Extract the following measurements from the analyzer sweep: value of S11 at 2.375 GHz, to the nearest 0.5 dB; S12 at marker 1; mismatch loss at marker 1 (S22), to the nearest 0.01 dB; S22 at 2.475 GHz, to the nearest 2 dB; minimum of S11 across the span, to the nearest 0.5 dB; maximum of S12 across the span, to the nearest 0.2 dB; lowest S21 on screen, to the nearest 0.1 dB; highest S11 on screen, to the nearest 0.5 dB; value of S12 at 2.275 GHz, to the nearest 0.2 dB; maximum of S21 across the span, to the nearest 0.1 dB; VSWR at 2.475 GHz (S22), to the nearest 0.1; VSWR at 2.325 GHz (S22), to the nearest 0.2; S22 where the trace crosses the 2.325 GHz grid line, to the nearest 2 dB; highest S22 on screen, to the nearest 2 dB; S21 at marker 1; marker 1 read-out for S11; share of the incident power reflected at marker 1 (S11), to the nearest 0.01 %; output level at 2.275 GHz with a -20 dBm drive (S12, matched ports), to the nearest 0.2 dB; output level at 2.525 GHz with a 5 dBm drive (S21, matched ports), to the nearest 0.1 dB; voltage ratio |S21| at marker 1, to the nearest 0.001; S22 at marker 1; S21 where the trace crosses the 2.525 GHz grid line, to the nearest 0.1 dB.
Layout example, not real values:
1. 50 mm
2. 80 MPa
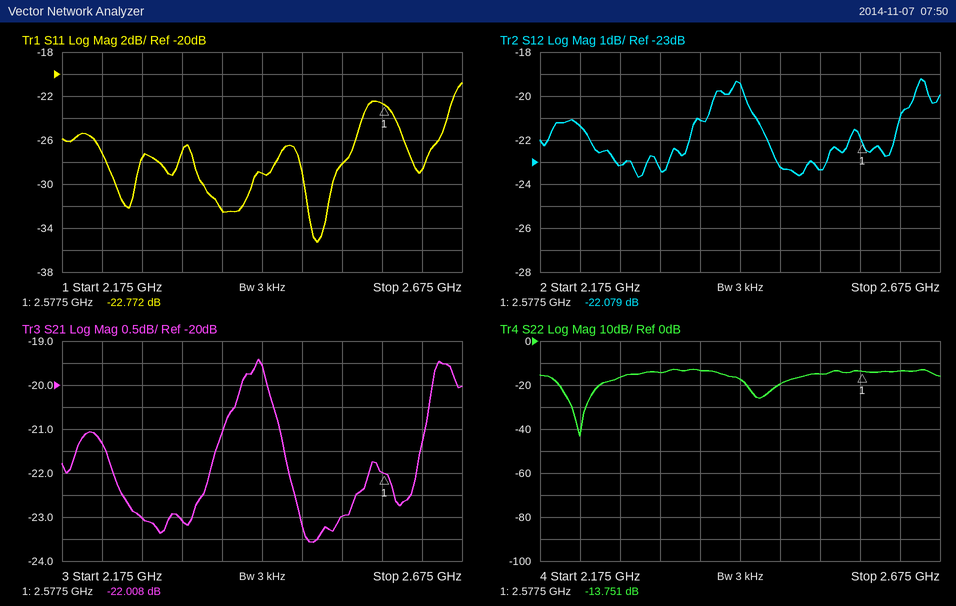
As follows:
1. -32.5 dB
2. -22.079 dB
3. 0.19 dB
4. -20 dB
5. -35.5 dB
6. -19.2 dB
7. -23.6 dB
8. -21.0 dB
9. -23.2 dB
10. -19.4 dB
11. 1.2
12. 1.4
13. -14 dB
14. -12 dB
15. -22.008 dB
16. -22.772 dB
17. 0.53 %
18. -43.2 dBm
19. -18.0 dBm
20. 0.079
21. -13.751 dB
22. -23.0 dB
